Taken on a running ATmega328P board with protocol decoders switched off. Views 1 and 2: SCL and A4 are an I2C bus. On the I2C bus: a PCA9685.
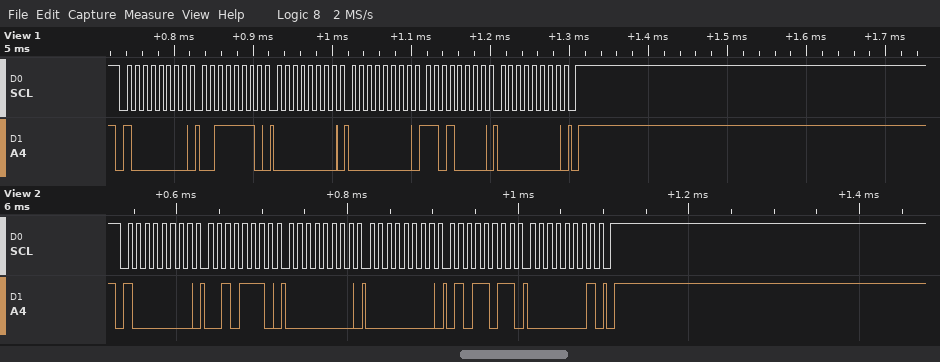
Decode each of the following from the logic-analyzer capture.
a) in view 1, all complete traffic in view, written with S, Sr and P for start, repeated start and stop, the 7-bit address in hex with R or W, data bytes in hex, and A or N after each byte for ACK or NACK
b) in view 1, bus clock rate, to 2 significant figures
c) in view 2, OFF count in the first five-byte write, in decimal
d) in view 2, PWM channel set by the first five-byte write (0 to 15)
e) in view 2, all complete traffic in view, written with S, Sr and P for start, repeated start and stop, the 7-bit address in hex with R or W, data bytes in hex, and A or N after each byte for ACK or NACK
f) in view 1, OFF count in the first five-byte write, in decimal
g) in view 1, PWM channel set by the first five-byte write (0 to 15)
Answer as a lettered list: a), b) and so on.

a) S 40W A 3E A 00 A 00 A D0 A 00 A P
b) 100 kHz
c) 347
d) 10
e) S 40W A 2E A 00 A 00 A 5B A 01 A P
f) 208
g) 14
